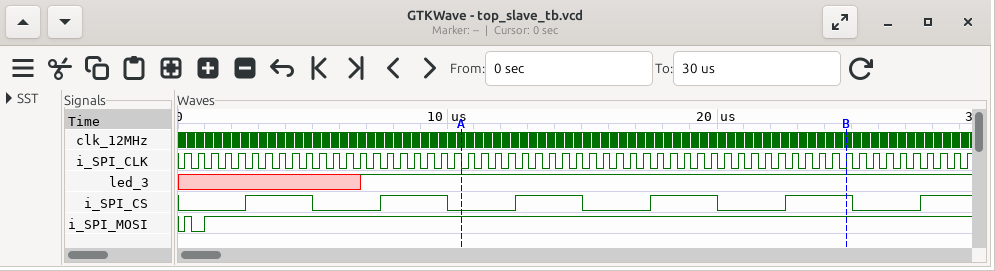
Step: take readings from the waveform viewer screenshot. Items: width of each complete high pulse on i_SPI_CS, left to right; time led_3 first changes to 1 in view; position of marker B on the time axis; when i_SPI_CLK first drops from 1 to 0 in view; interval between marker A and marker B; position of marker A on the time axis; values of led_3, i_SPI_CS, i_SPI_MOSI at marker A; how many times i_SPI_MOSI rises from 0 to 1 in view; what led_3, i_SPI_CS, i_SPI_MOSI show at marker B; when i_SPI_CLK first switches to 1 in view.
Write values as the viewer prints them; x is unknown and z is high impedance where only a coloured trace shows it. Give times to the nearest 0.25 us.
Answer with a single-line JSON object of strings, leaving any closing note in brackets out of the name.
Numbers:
{"width of each complete high pulse on i_SPI_CS, left to right": "2.5 us, 2.5 us, 2.5 us, 2.5 us, 2.5 us", "time led_3 first changes to 1 in view": "6.75 us", "position of marker B on the time axis": "24.75 us", "when i_SPI_CLK first drops from 1 to 0 in view": "0.5 us", "interval between marker A and marker B": "14.25 us", "position of marker A on the time axis": "10.5 us", "values of led_3, i_SPI_CS, i_SPI_MOSI at marker A": "led_3=1, i_SPI_CS=0, i_SPI_MOSI=1", "how many times i_SPI_MOSI rises from 0 to 1 in view": "2", "what led_3, i_SPI_CS, i_SPI_MOSI show at marker B": "led_3=1, i_SPI_CS=1, i_SPI_MOSI=1", "when i_SPI_CLK first switches to 1 in view": "0.25 us"}
